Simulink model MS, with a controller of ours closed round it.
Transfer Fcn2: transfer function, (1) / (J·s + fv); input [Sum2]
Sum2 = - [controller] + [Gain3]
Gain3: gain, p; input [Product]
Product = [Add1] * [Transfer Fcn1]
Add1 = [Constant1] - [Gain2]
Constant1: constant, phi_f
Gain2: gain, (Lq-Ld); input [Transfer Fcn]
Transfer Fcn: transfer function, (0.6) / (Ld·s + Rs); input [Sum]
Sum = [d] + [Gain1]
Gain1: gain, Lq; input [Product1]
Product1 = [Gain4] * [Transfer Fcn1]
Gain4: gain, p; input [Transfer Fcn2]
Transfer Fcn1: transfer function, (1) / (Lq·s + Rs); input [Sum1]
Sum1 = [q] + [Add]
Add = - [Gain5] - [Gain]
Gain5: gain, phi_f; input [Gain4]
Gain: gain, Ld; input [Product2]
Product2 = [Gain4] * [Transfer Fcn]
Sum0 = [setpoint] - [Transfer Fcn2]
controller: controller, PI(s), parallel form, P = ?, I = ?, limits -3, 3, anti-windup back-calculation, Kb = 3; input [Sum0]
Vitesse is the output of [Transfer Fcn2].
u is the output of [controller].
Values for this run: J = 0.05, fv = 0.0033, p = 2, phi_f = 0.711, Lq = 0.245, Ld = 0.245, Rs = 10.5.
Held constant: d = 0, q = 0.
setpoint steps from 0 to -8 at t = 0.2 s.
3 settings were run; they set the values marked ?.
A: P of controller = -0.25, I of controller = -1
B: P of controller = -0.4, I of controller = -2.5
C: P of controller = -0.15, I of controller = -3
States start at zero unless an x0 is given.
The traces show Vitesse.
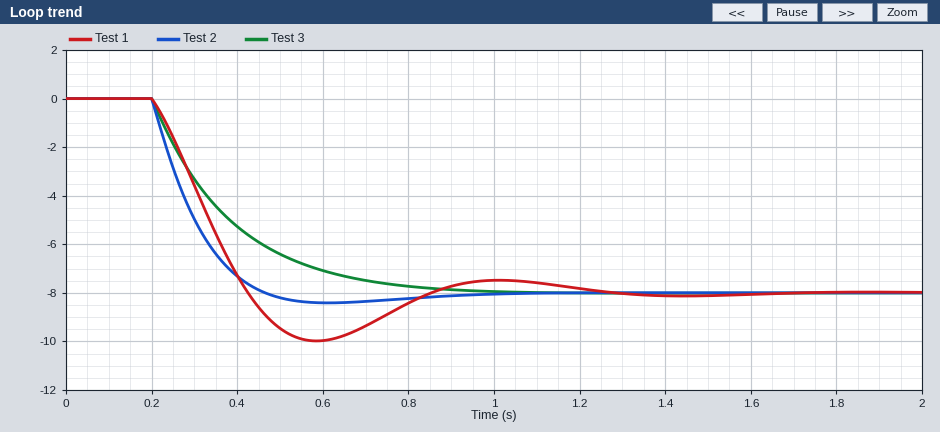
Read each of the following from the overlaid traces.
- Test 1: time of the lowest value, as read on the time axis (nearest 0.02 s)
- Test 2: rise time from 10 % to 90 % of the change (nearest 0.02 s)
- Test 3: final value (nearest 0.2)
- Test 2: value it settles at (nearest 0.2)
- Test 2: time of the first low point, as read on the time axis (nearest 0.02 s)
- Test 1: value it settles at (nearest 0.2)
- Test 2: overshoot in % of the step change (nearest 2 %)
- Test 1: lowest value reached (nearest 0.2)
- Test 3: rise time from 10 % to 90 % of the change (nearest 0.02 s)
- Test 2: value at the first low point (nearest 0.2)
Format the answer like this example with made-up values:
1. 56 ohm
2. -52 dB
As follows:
1. 0.58 s
2. 0.18 s
3. -8.0
4. -8.0
5. 0.62 s
6. -8.0
7. 6 %
8. -10.0
9. 0.40 s
10. -8.4
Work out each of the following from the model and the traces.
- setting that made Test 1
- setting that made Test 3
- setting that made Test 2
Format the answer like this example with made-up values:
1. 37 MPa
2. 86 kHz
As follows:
1. C
2. A
3. B
